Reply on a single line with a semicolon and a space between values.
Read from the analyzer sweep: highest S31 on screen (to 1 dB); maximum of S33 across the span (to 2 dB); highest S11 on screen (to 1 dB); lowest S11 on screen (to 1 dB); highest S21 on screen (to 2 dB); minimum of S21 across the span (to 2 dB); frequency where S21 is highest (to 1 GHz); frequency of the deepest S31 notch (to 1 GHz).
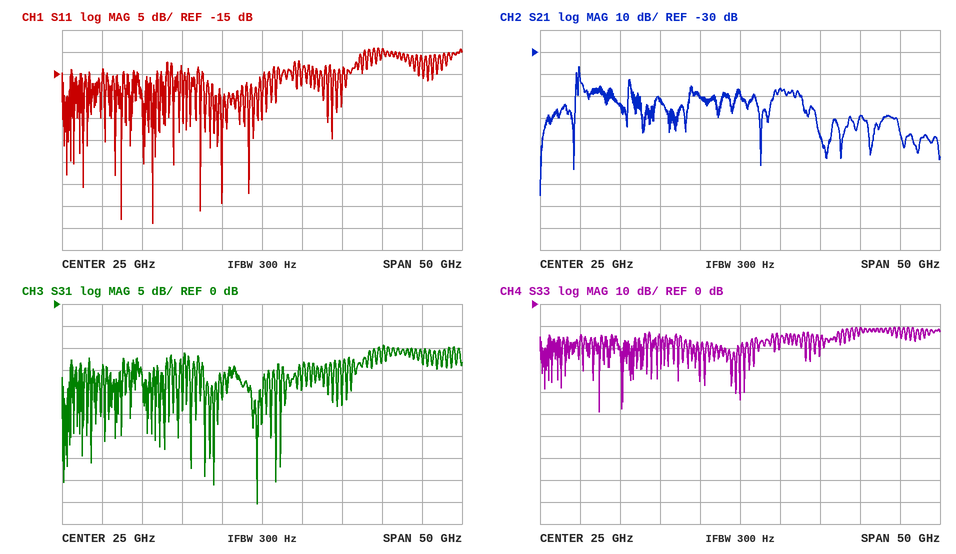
-9 dB; -10 dB; -9 dB; -49 dB; -36 dB; -96 dB; 5 GHz; 24 GHz
